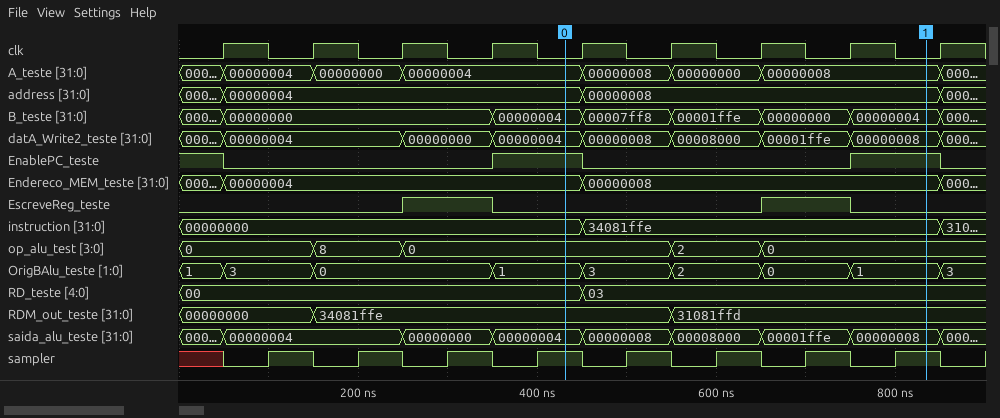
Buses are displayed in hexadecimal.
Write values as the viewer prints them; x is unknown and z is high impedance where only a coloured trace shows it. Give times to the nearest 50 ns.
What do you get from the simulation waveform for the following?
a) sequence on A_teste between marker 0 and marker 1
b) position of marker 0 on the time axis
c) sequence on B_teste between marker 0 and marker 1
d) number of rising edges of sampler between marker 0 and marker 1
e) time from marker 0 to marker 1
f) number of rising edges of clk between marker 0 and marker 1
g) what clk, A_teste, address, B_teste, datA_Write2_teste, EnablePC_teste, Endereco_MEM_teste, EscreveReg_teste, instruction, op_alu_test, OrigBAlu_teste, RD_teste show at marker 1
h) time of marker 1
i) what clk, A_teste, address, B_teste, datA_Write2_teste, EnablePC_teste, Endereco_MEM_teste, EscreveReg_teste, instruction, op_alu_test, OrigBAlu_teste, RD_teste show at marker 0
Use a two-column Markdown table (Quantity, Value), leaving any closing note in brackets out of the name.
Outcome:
| Quantity | Value |
|---|---|
| sequence on A_teste between marker 0 and marker 1 | 00000004, 00000008, 00000000, 00000008 |
| position of marker 0 on the time axis | 450 ns |
| sequence on B_teste between marker 0 and marker 1 | 00000004, 00007ff8, 00001ffe, 00000000, 00000004 |
| number of rising edges of sampler between marker 0 and marker 1 | 4 |
| time from marker 0 to marker 1 | 400 ns |
| number of rising edges of clk between marker 0 and marker 1 | 4 |
| what clk, A_teste, address, B_teste, datA_Write2_teste, EnablePC_teste, Endereco_MEM_teste, EscreveReg_teste, instruction, op_alu_test, OrigBAlu_teste, RD_teste show at marker 1 | clk=0, A_teste=00000008, address=00000008, B_teste=00000004, datA_Write2_teste=00000008, EnablePC_teste=1, Endereco_MEM_teste=00000008, EscreveReg_teste=0, instruction=34081ffe, op_alu_test=0, OrigBAlu_teste=1, RD_teste=03 |
| time of marker 1 | 850 ns |
| what clk, A_teste, address, B_teste, datA_Write2_teste, EnablePC_teste, Endereco_MEM_teste, EscreveReg_teste, instruction, op_alu_test, OrigBAlu_teste, RD_teste show at marker 0 | clk=0, A_teste=00000004, address=00000004, B_teste=00000004, datA_Write2_teste=00000004, EnablePC_teste=1, Endereco_MEM_teste=00000004, EscreveReg_teste=0, instruction=00000000, op_alu_test=0, OrigBAlu_teste=1, RD_teste=00 |
